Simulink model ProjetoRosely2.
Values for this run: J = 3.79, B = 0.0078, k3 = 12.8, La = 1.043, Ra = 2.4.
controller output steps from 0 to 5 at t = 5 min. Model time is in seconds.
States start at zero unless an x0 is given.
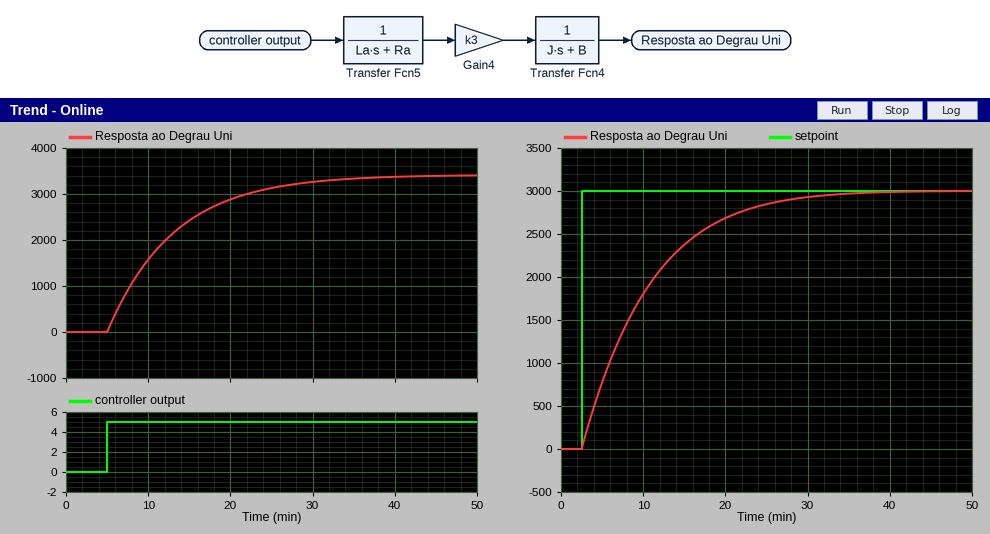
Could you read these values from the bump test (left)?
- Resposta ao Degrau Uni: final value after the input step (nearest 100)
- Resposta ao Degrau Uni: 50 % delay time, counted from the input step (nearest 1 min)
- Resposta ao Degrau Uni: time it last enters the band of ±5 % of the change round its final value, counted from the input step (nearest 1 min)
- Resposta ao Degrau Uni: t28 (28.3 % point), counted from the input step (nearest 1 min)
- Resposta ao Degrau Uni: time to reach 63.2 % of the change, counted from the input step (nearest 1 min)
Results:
3400
6 min
24 min
3 min
8 min
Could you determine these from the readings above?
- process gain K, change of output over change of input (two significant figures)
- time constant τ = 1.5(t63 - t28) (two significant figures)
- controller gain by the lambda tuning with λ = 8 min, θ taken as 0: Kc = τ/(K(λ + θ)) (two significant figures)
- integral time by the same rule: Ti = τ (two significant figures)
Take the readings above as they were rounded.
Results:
680
7.5 min
0.0014
7.5 min
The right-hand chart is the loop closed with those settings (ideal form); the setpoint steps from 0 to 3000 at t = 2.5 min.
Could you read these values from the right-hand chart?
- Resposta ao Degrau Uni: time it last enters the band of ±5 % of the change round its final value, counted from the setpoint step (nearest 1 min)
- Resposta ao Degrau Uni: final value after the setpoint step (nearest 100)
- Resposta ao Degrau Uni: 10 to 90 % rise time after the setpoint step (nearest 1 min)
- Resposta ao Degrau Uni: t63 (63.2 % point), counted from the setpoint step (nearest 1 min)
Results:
23 min
3000
17 min
8 min
